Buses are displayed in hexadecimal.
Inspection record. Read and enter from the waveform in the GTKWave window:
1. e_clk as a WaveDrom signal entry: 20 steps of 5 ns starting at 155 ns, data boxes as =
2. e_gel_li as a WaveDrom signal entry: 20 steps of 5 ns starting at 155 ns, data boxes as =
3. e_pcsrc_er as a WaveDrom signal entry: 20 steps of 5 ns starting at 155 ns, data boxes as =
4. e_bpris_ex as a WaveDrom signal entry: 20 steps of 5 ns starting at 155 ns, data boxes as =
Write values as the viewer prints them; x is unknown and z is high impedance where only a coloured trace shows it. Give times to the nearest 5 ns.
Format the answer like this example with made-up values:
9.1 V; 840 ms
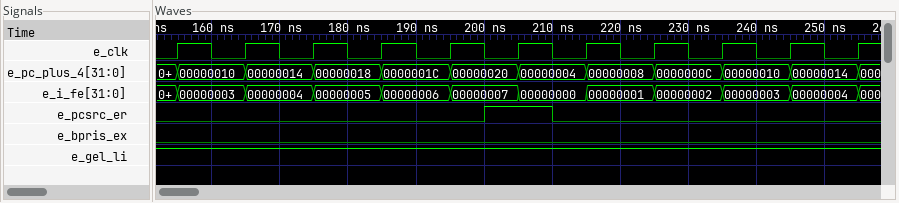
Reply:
{name: 'e_clk', wave: '10101010101010101010'}; {name: 'e_gel_li', wave: '1...................'}; {name: 'e_pcsrc_er', wave: '0........1.0........'}; {name: 'e_bpris_ex', wave: '0...................'}
